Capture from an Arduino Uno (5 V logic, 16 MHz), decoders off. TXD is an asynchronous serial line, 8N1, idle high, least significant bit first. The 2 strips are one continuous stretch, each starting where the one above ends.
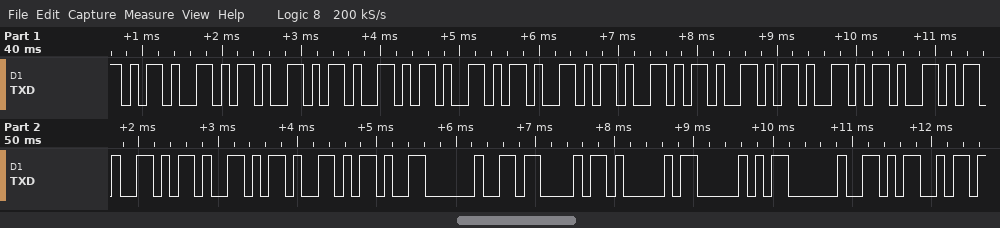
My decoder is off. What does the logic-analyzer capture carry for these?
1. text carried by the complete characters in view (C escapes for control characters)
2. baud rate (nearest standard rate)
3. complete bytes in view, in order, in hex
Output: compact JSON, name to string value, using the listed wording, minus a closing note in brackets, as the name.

{"text carried by the complete characters in view": "\"------------- CAP M\"", "baud rate": "9600 baud", "complete bytes in view, in order, in hex": "2D 2D 2D 2D 2D 2D 2D 2D 2D 2D 2D 2D 2D 20 43 41 50 20 4D"}
